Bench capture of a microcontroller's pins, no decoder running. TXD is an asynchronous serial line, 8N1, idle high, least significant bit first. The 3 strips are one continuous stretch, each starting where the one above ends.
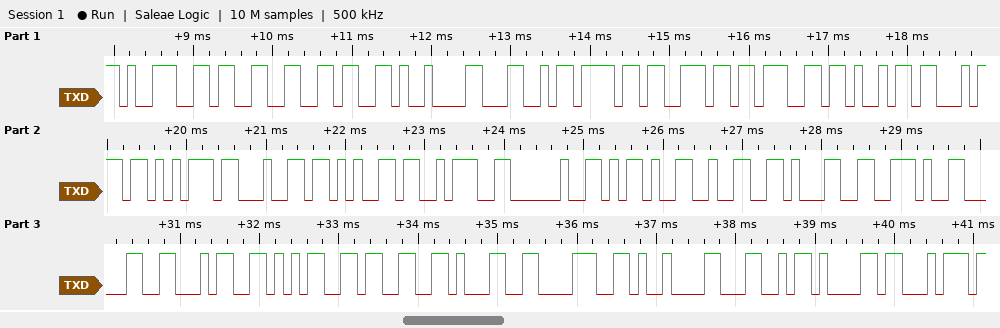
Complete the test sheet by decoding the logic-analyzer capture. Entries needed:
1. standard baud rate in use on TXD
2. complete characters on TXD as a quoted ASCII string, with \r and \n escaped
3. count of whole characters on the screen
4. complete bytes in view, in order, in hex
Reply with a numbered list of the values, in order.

1. 9600 baud
2. "936\tLongitude: -21.045318\tLat"
3. 29
4. 39 33 36 09 4C 6F 6E 67 69 74 75 64 65 3A 20 2D 32 31 2E 30 34 35 33 31 38 09 4C 61 74
